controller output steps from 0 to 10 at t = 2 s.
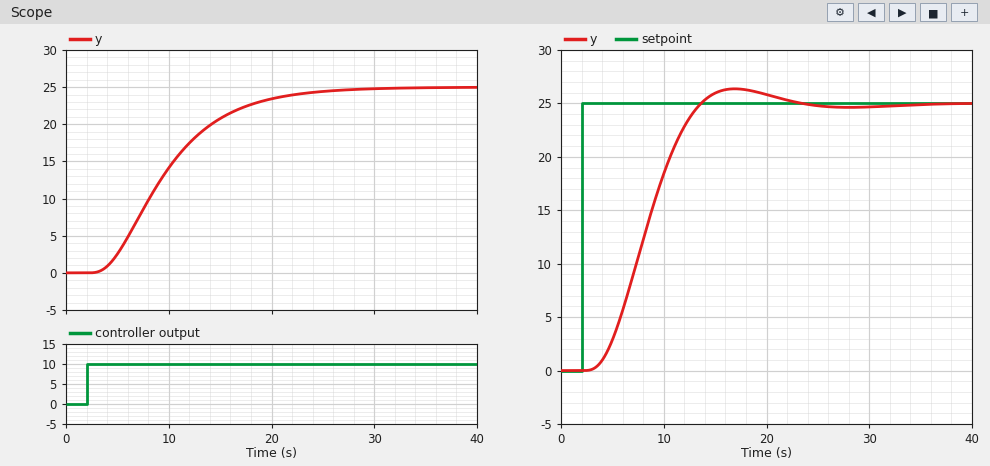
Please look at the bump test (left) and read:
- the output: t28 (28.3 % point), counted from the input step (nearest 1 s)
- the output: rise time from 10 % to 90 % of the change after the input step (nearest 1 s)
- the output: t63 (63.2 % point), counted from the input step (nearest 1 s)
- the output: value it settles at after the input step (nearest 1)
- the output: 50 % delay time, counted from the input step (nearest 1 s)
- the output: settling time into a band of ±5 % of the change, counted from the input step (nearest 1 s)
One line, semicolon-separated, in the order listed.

5 s; 13 s; 9 s; 25; 7 s; 19 s
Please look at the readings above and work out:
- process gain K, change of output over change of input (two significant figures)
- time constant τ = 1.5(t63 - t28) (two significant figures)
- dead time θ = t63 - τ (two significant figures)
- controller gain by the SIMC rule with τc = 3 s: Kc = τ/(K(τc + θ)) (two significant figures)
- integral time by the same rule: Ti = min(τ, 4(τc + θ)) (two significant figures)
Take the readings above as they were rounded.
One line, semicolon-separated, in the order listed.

2.5; 6.0 s; 3.0 s; 0.40; 6.0 s
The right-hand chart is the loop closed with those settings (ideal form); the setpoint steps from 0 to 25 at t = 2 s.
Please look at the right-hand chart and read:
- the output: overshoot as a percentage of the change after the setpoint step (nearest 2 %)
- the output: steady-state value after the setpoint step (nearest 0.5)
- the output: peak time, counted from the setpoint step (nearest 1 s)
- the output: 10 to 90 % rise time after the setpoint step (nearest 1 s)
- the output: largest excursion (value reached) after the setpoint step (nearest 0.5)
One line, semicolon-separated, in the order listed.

6 %; 25.0; 15 s; 7 s; 26.5
